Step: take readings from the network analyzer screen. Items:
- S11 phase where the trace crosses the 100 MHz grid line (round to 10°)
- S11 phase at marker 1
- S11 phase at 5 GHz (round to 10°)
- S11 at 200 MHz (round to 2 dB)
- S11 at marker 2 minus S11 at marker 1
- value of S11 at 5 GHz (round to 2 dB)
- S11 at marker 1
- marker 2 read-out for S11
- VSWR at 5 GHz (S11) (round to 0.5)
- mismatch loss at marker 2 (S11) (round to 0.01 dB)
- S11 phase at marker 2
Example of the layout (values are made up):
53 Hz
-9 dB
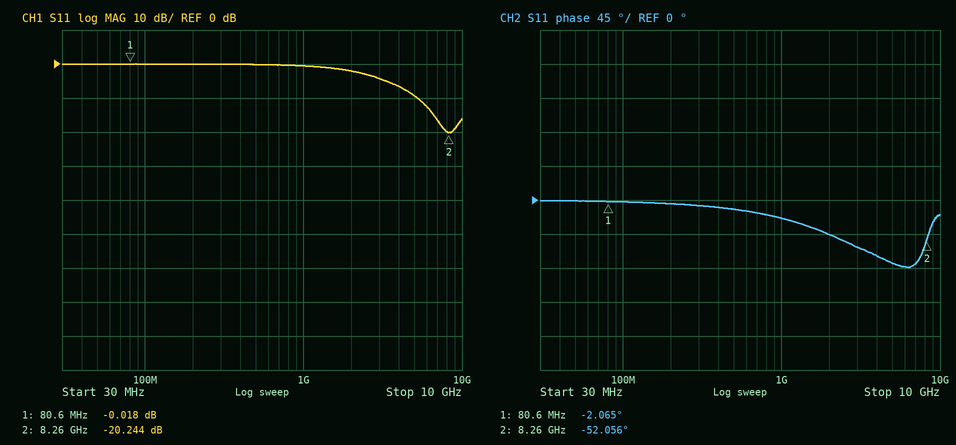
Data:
0°
-2.065°
-80°
0 dB
-20.226 dB
-10 dB
-0.018 dB
-20.244 dB
2.0
0.04 dB
-52.056°
